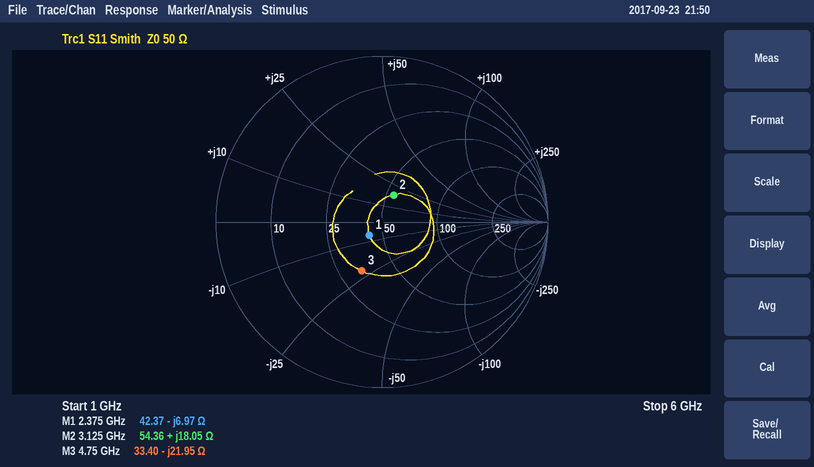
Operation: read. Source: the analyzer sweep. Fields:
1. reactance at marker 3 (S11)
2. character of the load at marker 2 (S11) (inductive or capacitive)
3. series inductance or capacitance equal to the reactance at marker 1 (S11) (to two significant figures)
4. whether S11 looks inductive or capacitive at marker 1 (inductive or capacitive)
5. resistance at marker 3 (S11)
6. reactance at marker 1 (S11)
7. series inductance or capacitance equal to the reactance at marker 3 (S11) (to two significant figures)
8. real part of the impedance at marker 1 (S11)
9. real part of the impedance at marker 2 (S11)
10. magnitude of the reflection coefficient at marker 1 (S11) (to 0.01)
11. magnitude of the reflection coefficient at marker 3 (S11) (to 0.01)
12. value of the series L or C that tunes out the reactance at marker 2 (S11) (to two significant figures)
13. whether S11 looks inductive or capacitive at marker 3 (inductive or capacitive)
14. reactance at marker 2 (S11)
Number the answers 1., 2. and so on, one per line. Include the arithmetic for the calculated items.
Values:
1. -21.95 Ω
2. inductive
3. C = 1/(2π × 2.375 GHz × 6.97 Ω) ≈ 9.6 pF
4. capacitive
5. 33.40 Ω
6. -6.97 Ω
7. C = 1/(2π × 4.75 GHz × 21.95 Ω) ≈ 1.5 pF
8. 42.37 Ω
9. 54.36 Ω
10. 0.11
11. 0.32
12. C = 1/(2π × 3.125 GHz × 18.05 Ω) ≈ 2.8 pF
13. capacitive
14. +18.05 Ω
